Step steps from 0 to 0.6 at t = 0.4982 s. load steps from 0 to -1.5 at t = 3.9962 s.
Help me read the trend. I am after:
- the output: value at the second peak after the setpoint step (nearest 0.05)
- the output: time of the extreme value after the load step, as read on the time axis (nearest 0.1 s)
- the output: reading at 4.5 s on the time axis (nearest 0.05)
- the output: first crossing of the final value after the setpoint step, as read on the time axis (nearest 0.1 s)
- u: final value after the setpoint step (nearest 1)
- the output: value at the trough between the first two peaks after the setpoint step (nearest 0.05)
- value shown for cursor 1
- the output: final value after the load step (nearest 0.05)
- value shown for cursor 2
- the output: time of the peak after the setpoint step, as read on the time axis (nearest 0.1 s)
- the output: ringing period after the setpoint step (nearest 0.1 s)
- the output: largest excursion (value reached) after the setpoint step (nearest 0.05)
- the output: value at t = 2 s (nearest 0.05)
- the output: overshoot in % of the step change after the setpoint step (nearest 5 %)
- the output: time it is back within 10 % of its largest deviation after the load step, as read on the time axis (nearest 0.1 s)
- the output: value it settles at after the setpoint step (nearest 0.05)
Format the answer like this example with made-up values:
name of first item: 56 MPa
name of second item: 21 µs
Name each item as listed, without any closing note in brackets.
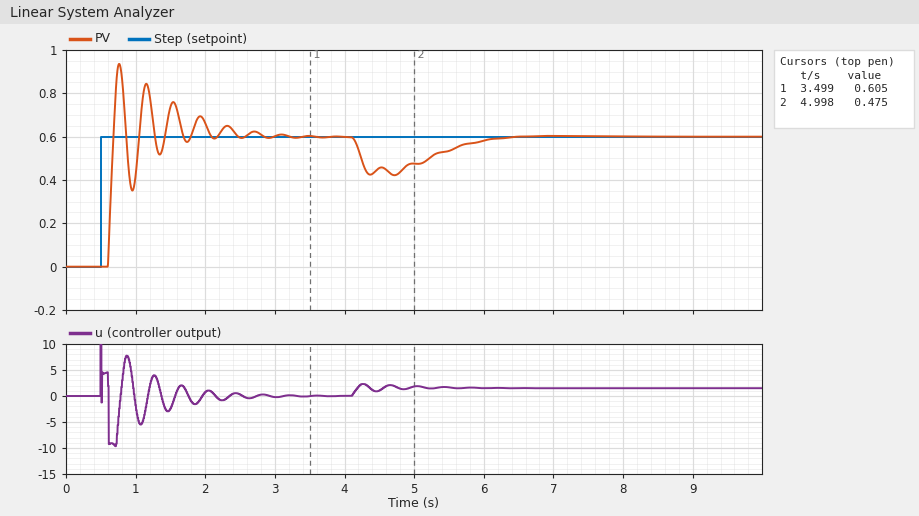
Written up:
the output: value at the second peak after the setpoint step: 0.85
the output: time of the extreme value after the load step, as read on the time axis: 4.7 s
the output: reading at 4.5 s on the time axis: 0.45
the output: first crossing of the final value after the setpoint step, as read on the time axis: 0.7 s
u: final value after the setpoint step: 0
the output: value at the trough between the first two peaks after the setpoint step: 0.35
value shown for cursor 1: 0.605
the output: final value after the load step: 0.60
value shown for cursor 2: 0.475
the output: time of the peak after the setpoint step, as read on the time axis: 0.8 s
the output: ringing period after the setpoint step: 0.4 s
the output: largest excursion (value reached) after the setpoint step: 0.95
the output: value at t = 2 s: 0.65
the output: overshoot in % of the step change after the setpoint step: 55 %
the output: time it is back within 10 % of its largest deviation after the load step, as read on the time axis: 6.0 s
the output: value it settles at after the setpoint step: 0.60
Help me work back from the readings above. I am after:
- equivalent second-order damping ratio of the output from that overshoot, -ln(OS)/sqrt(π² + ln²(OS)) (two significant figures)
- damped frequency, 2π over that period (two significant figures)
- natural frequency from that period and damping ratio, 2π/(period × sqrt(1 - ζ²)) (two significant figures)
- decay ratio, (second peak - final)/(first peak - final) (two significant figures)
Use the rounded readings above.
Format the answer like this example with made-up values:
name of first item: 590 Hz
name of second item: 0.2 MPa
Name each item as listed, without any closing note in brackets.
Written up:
equivalent second-order damping ratio of the output from that overshoot, -ln(OS)/sqrt(π² + ln²(OS)): 0.19
damped frequency, 2π over that period: 16 rad/s
natural frequency from that period and damping ratio, 2π/(period × sqrt(1 - ζ²)): 16 rad/s
decay ratio, (second peak - final)/(first peak - final): 0.71
